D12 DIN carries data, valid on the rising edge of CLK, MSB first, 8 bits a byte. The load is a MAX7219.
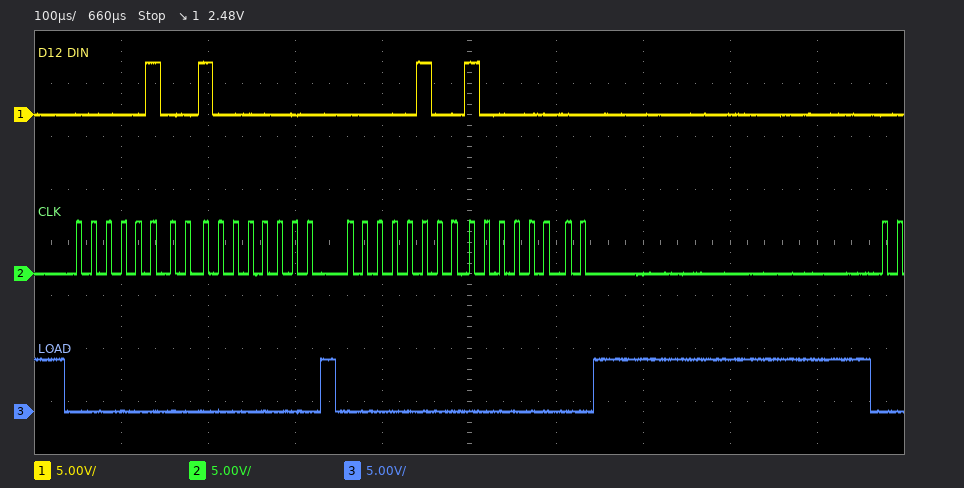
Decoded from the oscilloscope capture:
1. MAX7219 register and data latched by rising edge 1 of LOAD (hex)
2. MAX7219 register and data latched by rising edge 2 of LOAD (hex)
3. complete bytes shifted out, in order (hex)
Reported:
register 0x4, data 0x80
register 0x4, data 0x80
04 80 04 80
